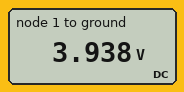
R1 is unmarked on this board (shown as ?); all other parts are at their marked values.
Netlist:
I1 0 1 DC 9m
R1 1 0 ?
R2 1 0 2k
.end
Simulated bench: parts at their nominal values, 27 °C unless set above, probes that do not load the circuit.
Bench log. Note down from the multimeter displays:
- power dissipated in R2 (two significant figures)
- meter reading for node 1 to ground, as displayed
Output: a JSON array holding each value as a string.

["7.8 mW", "3.938 V"]
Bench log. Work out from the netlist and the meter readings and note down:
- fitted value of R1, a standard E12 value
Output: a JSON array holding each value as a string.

["560 Ω"]
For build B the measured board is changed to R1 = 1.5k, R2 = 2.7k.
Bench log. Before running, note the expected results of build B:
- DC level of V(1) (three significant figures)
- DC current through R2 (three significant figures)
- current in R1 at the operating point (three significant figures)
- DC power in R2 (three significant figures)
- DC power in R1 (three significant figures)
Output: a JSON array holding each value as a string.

["8.68 V", "3.21 mA", "5.79 mA", "27.9 mW", "50.2 mW"]
